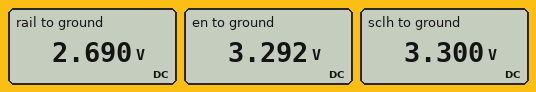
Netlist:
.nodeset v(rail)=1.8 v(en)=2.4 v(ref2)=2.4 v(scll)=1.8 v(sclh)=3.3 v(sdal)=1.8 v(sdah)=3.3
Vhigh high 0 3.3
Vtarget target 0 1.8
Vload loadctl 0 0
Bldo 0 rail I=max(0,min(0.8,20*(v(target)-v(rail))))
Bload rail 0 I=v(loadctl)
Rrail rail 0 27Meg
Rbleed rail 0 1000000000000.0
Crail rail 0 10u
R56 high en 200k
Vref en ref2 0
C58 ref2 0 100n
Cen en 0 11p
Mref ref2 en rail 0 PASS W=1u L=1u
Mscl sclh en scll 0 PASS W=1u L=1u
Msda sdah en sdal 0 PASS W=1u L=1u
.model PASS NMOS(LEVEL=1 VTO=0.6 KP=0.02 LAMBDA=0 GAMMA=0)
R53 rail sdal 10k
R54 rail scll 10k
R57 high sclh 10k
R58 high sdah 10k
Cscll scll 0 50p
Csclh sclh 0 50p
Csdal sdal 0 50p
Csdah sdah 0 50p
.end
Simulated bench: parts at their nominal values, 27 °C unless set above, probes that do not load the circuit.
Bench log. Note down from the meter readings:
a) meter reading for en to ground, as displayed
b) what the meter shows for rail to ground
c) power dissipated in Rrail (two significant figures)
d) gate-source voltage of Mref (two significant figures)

3.292 V
2.690 V
270 nW
600 mV
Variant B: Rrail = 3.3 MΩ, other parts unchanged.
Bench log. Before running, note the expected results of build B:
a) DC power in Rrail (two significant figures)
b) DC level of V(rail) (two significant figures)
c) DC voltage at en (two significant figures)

2.1 µW
2.6 V
3.2 V
